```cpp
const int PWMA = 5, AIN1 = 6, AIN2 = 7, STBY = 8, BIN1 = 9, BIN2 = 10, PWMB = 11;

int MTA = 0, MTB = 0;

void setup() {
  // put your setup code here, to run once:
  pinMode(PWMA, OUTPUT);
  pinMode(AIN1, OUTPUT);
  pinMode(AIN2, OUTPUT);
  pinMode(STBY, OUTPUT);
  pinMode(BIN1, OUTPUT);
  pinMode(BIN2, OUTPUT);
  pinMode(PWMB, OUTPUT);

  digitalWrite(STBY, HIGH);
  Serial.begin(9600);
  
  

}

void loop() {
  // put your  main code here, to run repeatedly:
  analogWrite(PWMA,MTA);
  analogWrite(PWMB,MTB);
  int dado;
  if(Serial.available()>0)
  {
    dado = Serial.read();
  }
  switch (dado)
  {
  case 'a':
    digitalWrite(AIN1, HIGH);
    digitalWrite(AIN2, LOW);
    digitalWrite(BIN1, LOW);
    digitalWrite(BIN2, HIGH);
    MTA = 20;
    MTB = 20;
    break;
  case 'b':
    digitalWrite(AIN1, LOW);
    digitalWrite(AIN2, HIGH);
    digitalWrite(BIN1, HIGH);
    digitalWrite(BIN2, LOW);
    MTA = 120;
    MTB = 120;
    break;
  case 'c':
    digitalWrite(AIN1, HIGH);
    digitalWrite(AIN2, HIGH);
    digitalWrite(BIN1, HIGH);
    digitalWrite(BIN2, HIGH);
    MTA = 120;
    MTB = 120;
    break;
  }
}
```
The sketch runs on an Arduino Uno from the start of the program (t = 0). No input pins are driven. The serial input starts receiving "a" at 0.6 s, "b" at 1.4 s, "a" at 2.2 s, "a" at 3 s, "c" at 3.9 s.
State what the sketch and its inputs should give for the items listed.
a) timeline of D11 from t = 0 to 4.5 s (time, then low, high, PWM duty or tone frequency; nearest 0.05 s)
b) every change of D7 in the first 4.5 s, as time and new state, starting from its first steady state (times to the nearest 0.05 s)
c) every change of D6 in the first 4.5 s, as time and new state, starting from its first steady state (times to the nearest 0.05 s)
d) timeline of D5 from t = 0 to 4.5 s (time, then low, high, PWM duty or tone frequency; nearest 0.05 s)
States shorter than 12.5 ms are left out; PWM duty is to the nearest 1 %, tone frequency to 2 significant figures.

0 s low; 0.6 s PWM 8 %; 1.4 s PWM 47 %; 2.2 s PWM 8 %; 3.9 s PWM 47 %
0 s low; 1.4 s high; 2.2 s low; 3.9 s high
0 s low; 0.6 s high; 1.4 s low; 2.2 s high
0 s low; 0.6 s PWM 8 %; 1.4 s PWM 47 %; 2.2 s PWM 8 %; 3.9 s PWM 47 %
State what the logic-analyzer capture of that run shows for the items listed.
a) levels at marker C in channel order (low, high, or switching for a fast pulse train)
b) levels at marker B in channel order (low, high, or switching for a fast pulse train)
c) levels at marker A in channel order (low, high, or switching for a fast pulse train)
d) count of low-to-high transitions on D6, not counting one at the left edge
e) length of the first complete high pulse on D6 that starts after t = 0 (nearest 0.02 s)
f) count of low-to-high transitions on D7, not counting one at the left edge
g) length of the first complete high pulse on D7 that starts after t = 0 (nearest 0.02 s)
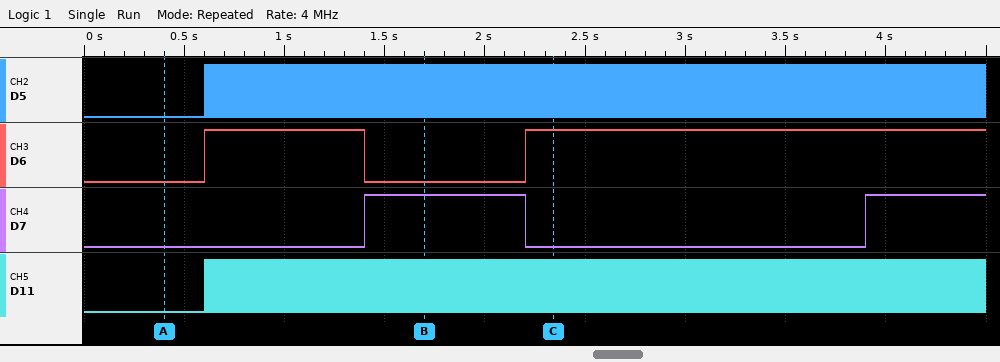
D5 switching, D6 high, D7 low, D11 switching
D5 switching, D6 low, D7 high, D11 switching
D5 low, D6 low, D7 low, D11 low
2
0.80 s
2
0.80 s
